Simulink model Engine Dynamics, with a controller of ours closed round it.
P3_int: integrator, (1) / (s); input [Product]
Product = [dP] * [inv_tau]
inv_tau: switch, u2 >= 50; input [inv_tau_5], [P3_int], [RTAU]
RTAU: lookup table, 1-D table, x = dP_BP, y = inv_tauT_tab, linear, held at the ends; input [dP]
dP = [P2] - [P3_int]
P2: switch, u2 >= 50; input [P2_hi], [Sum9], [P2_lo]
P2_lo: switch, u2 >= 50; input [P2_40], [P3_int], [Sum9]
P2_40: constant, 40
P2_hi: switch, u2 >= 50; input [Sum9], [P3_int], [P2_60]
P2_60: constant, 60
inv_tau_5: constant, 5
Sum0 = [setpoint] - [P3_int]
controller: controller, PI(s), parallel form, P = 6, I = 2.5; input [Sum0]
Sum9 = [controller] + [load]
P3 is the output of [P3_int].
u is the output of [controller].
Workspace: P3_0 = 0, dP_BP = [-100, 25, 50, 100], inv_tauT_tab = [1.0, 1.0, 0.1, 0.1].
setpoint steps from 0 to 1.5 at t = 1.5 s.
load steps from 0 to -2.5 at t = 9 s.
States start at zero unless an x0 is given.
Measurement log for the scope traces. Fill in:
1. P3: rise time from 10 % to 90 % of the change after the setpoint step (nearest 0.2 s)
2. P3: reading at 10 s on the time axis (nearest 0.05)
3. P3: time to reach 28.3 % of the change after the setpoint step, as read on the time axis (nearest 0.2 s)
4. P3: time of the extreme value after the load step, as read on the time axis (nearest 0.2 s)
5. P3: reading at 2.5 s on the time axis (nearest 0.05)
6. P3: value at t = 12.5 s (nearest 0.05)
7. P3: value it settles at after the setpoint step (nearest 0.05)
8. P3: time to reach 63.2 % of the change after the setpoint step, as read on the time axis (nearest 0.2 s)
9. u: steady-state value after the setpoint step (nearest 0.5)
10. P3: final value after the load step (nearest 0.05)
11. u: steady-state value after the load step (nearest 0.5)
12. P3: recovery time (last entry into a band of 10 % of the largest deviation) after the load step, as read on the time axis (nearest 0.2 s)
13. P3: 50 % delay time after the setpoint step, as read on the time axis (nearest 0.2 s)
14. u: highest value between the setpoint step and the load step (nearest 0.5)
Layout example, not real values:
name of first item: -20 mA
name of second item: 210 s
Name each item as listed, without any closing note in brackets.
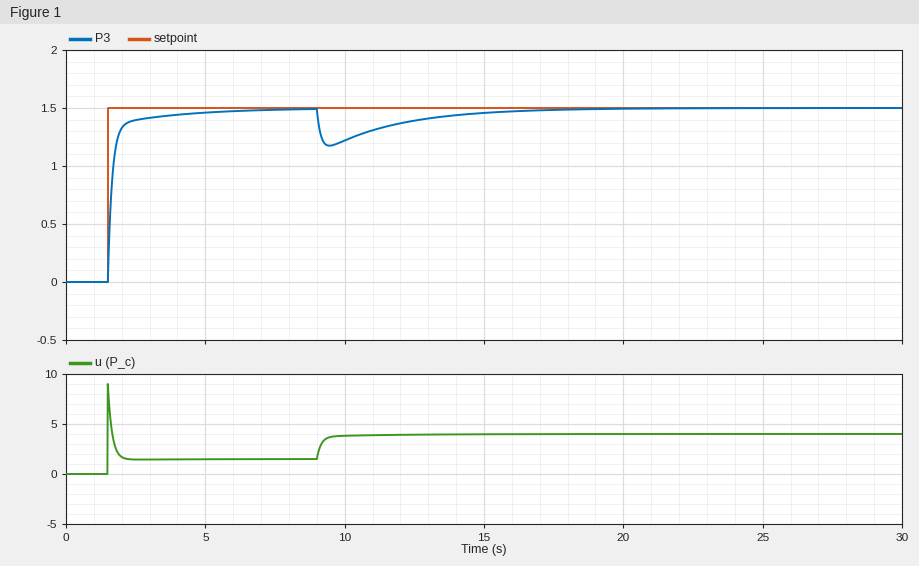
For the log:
P3: rise time from 10 % to 90 % of the change after the setpoint step: 0.6 s
P3: reading at 10 s on the time axis: 1.20
P3: time to reach 28.3 % of the change after the setpoint step, as read on the time axis: 1.6 s
P3: time of the extreme value after the load step, as read on the time axis: 9.4 s
P3: reading at 2.5 s on the time axis: 1.40
P3: value at t = 12.5 s: 1.40
P3: value it settles at after the setpoint step: 1.50
P3: time to reach 63.2 % of the change after the setpoint step, as read on the time axis: 1.6 s
u: steady-state value after the setpoint step: 1.5
P3: final value after the load step: 1.50
u: steady-state value after the load step: 4.0
P3: recovery time (last entry into a band of 10 % of the largest deviation) after the load step, as read on the time axis: 15.8 s
P3: 50 % delay time after the setpoint step, as read on the time axis: 1.6 s
u: highest value between the setpoint step and the load step: 9.0
